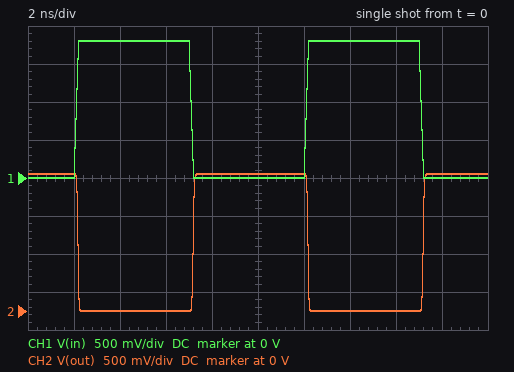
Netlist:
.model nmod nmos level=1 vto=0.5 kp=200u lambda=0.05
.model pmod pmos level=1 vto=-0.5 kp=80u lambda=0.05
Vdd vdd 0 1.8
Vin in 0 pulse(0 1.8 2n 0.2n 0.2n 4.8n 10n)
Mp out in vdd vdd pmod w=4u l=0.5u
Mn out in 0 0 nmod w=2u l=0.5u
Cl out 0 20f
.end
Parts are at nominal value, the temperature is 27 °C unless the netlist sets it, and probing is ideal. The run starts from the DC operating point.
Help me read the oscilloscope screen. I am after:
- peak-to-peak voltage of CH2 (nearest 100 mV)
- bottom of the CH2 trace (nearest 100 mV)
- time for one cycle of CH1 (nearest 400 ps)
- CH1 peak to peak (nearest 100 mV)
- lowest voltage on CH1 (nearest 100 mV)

1.8 V
0 V
10.0 ns
1.8 V
0 V
